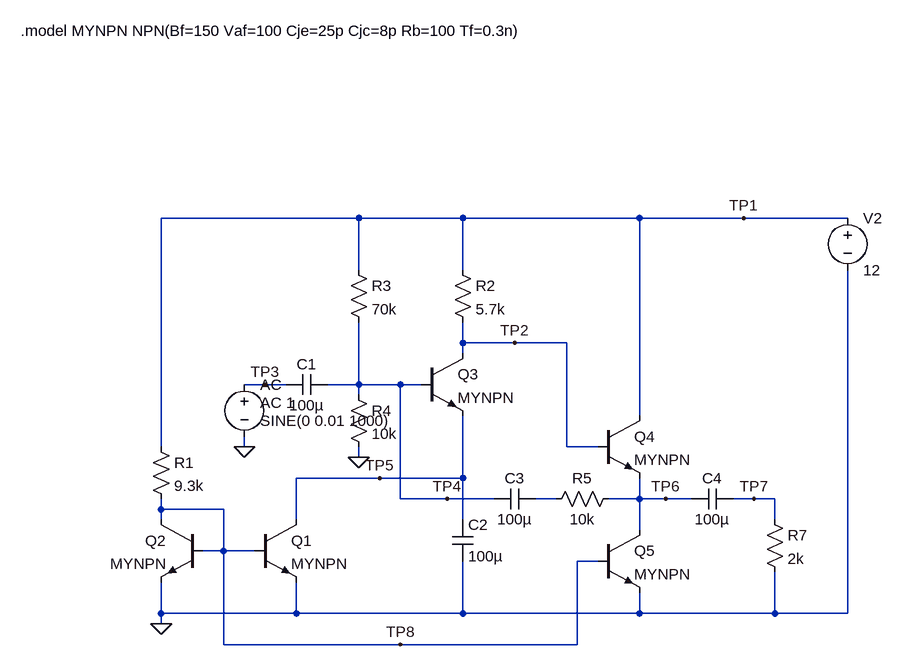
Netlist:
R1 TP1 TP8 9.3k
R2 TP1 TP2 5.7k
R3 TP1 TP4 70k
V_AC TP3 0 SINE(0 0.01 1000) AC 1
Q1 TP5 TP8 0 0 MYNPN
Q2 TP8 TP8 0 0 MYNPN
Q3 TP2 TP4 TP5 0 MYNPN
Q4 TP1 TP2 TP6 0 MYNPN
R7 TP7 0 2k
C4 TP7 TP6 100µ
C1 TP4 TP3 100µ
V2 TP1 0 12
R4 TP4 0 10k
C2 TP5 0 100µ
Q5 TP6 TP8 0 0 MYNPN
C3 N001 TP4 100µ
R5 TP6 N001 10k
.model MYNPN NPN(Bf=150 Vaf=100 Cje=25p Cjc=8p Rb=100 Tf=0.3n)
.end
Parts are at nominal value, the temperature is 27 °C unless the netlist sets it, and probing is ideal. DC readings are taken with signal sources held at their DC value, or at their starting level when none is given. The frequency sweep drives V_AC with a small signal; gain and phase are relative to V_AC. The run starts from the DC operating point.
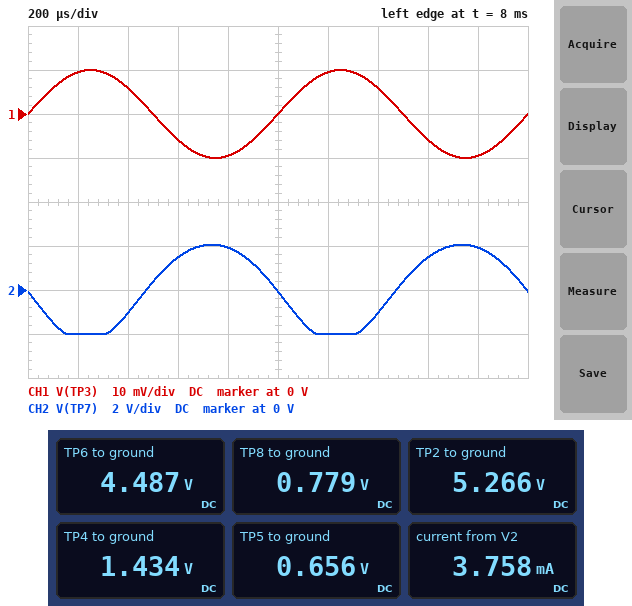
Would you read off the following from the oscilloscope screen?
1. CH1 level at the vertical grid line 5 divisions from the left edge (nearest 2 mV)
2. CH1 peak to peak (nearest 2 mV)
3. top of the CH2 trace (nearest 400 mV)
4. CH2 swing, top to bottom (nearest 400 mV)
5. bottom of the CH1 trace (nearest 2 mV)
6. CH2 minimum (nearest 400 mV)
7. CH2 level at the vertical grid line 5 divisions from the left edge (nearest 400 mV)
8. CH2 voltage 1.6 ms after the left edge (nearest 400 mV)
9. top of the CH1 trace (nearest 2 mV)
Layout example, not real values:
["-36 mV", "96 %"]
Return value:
["0 V", "20 mV", "2.0 V", "4.0 V", "-10 mV", "-2.0 V", "0 V", "1.6 V", "10 mV"]
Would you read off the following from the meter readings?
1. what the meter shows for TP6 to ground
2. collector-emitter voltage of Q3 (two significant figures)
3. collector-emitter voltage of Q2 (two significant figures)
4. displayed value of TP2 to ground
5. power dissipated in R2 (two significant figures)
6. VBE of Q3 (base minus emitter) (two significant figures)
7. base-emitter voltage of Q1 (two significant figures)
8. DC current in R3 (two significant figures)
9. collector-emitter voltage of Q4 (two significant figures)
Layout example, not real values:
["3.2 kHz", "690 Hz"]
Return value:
["4.487 V", "4.6 V", "780 mV", "5.266 V", "8.0 mW", "780 mV", "780 mV", "150 µA", "7.5 V"]
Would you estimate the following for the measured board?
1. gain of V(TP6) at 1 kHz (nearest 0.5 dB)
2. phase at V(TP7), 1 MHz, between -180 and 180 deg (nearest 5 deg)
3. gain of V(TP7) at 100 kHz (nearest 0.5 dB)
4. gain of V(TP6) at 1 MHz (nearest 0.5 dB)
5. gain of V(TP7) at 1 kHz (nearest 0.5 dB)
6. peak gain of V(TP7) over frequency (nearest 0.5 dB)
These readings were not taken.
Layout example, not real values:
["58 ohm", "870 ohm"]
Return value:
["47.0 dB", "135 deg", "47.0 dB", "44.5 dB", "47.0 dB", "47.0 dB"]
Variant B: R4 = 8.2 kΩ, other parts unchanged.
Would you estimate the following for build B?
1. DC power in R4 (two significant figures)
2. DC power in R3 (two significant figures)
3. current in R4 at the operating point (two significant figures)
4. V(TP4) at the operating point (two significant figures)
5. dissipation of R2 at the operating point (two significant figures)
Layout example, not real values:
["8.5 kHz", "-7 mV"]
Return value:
["180 µW", "1.7 mW", "150 µA", "1.2 V", "7.9 mW"]
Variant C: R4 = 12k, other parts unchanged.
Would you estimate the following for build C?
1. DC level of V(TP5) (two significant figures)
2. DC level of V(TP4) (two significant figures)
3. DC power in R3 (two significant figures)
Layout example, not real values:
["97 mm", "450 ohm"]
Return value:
["900 mV", "1.7 V", "1.5 mW"]
